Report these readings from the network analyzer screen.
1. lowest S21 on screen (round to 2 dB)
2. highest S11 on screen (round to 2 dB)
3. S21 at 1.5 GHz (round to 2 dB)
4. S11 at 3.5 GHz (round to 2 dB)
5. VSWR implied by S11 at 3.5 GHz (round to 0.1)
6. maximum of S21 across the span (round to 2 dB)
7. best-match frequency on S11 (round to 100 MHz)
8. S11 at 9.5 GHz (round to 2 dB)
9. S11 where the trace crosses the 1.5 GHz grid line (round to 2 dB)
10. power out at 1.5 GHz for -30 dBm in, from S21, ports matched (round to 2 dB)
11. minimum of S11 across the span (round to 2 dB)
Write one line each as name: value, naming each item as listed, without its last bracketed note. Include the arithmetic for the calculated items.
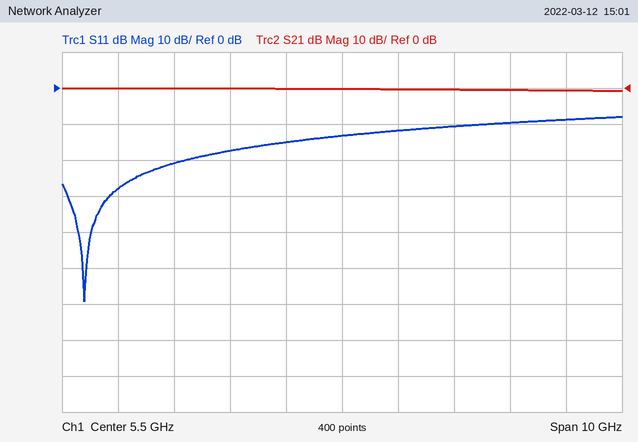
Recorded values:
lowest S21 on screen: 0 dB
highest S11 on screen: -8 dB
S21 at 1.5 GHz: 0 dB
S11 at 3.5 GHz: -18 dB
VSWR implied by S11 at 3.5 GHz: |Γ| = 10^(-18/20) = 0.1259; VSWR = (1 + 0.1259)/(1 − 0.1259) ≈ 1.3
maximum of S21 across the span: 0 dB
best-match frequency on S11: 900 MHz
S11 at 9.5 GHz: -8 dB
S11 where the trace crosses the 1.5 GHz grid line: -28 dB
power out at 1.5 GHz for -30 dBm in, from S21, ports matched: -30 dBm + (0 dB) = -30 dBm
minimum of S11 across the span: -60 dB
